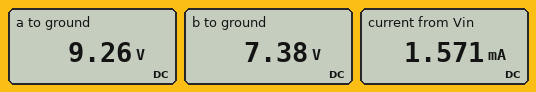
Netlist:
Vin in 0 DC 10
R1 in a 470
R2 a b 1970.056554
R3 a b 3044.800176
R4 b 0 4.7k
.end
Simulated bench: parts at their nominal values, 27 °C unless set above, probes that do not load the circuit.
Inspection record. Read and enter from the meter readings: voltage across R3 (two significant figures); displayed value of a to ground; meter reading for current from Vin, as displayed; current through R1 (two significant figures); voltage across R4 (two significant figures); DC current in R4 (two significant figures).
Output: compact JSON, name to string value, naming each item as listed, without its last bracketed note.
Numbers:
{"voltage across R3": "1.9 V", "displayed value of a to ground": "9.26 V", "meter reading for current from Vin, as displayed": "1.571 mA", "current through R1": "1.6 mA", "voltage across R4": "7.4 V", "DC current in R4": "1.6 mA"}
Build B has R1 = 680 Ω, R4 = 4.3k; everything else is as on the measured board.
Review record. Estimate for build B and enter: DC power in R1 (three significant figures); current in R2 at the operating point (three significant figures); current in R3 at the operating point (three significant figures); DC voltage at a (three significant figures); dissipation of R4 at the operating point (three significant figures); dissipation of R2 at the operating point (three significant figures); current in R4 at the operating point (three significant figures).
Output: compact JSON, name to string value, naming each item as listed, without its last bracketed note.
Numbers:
{"DC power in R1": "1.78 mW", "current in R2 at the operating point": "983 µA", "current in R3 at the operating point": "636 µA", "DC voltage at a": "8.90 V", "dissipation of R4 at the operating point": "11.3 mW", "dissipation of R2 at the operating point": "1.90 mW", "current in R4 at the operating point": "1.62 mA"}
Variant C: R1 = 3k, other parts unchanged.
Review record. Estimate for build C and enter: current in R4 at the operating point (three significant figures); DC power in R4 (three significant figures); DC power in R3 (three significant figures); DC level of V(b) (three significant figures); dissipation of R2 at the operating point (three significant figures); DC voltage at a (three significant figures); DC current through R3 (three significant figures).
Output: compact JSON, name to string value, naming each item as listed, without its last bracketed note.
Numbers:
{"current in R4 at the operating point": "1.12 mA", "DC power in R4": "5.94 mW", "DC power in R3": "594 µW", "DC level of V(b)": "5.28 V", "dissipation of R2 at the operating point": "918 µW", "DC voltage at a": "6.63 V", "DC current through R3": "442 µA"}
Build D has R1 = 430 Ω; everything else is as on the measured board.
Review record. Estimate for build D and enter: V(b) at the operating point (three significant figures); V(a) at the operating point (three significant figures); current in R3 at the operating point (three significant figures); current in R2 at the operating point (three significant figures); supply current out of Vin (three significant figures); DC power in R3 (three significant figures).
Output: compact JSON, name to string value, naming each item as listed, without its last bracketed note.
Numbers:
{"V(b) at the operating point": "7.43 V", "V(a) at the operating point": "9.32 V", "current in R3 at the operating point": "621 µA", "current in R2 at the operating point": "960 µA", "supply current out of Vin": "1.58 mA", "DC power in R3": "1.17 mW"}
